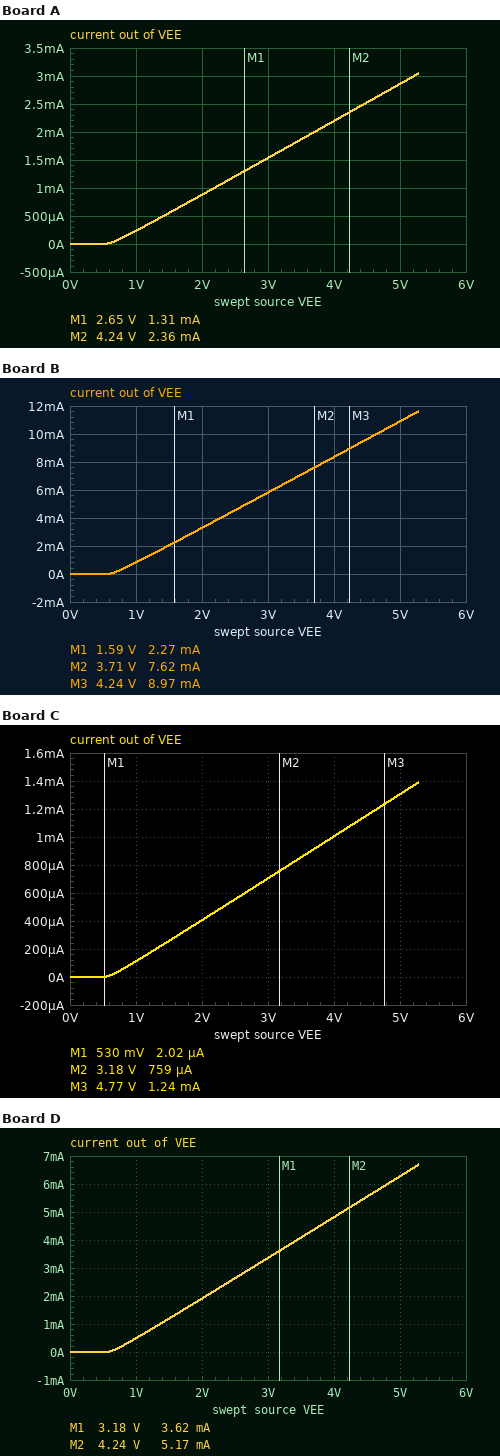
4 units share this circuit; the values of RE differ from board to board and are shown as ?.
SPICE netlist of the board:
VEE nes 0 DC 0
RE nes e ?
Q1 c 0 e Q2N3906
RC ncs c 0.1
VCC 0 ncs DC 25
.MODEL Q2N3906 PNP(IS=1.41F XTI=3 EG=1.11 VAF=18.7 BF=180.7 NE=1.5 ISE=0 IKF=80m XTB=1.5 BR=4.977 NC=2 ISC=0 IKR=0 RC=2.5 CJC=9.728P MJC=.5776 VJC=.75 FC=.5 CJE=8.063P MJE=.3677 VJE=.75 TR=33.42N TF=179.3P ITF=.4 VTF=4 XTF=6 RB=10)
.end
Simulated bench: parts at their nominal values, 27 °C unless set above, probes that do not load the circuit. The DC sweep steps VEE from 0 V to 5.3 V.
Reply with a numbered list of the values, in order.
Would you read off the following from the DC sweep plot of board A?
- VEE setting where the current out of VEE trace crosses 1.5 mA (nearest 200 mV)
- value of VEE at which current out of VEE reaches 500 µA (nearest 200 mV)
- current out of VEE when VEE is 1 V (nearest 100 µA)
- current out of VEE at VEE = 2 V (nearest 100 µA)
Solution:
1. 3.0 V
2. 1.4 V
3. 200 µA
4. 900 µA
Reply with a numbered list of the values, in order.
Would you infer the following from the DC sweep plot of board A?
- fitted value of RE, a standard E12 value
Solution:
1. 1.5 kΩ
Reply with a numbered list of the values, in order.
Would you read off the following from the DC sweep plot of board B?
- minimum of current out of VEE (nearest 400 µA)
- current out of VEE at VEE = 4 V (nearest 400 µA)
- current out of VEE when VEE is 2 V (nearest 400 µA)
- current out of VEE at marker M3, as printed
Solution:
1. 0 A
2. 8.4 mA
3. 3.2 mA
4. 8.97 mA
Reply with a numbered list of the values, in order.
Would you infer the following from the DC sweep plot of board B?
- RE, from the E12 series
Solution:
1. 390 Ω
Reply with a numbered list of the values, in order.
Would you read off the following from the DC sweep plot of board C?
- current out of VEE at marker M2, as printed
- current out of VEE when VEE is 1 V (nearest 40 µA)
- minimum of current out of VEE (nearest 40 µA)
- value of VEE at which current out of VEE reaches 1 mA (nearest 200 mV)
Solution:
1. 759 µA
2. 120 µA
3. 0 A
4. 4.0 V
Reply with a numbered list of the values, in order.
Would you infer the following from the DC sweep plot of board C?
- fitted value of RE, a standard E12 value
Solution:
1. 3.3 kΩ
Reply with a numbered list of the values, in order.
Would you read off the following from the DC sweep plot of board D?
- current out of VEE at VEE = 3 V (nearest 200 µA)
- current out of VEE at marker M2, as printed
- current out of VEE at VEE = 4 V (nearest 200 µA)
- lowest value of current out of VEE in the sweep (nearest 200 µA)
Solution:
1. 3.4 mA
2. 5.17 mA
3. 4.8 mA
4. 0 A
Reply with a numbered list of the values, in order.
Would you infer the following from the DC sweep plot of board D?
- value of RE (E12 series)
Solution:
1. 680 Ω
